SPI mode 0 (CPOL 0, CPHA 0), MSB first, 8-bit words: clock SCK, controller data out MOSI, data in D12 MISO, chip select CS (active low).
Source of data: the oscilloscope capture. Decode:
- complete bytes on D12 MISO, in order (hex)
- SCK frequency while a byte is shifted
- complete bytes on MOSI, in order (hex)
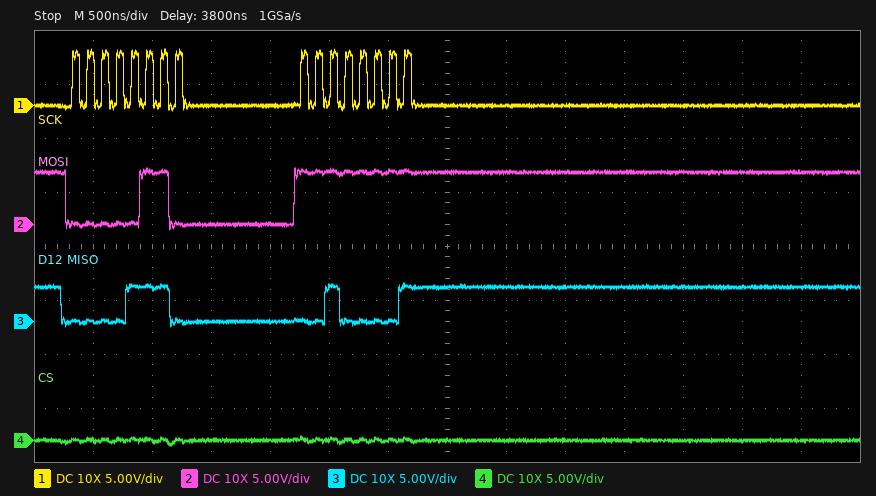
0x0E 0x21
8 MHz
0x06 0xFF
